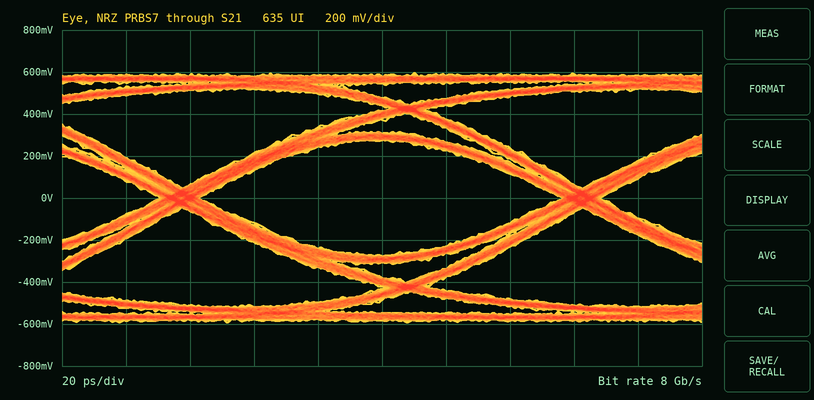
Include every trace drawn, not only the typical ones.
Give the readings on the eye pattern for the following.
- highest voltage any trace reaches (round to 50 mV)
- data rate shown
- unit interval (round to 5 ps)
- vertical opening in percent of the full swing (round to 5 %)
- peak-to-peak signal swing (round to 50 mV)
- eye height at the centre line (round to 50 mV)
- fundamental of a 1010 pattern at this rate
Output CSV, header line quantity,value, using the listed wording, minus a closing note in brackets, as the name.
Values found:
quantity,value
highest voltage any trace reaches,600 mV
data rate shown,8 Gb/s
unit interval,125 ps
vertical opening in percent of the full swing,45 %
peak-to-peak signal swing,1.20 V
eye height at the centre line,550 mV
fundamental of a 1010 pattern at this rate,4 GHz
